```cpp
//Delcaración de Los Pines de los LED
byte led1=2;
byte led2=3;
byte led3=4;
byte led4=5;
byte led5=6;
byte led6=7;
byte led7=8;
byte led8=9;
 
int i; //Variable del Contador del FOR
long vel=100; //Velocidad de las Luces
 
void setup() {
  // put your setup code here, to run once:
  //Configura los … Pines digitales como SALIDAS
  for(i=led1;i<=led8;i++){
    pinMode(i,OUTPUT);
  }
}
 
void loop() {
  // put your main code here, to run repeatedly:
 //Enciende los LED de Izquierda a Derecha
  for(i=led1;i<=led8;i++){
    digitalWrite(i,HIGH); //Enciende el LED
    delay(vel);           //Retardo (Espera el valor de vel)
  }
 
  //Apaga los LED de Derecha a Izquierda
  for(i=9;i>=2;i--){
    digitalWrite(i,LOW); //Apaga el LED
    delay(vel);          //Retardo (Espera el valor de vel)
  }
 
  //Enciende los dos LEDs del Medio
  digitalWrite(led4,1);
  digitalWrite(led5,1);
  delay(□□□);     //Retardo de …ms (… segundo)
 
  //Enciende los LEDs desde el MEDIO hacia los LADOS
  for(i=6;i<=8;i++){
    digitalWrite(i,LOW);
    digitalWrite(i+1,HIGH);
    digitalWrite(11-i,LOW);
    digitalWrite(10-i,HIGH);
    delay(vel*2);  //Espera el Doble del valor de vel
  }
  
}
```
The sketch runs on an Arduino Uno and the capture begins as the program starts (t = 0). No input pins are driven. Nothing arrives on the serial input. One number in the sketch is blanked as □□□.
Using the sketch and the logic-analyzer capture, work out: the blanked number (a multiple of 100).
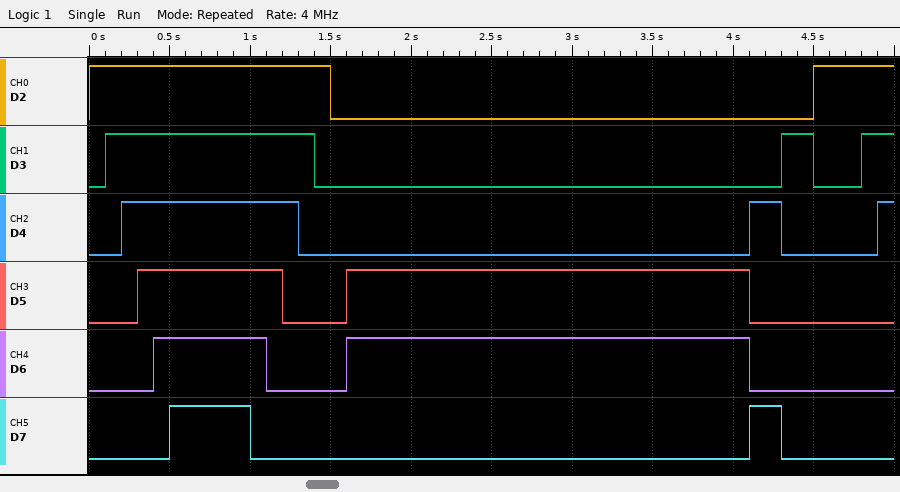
2500
